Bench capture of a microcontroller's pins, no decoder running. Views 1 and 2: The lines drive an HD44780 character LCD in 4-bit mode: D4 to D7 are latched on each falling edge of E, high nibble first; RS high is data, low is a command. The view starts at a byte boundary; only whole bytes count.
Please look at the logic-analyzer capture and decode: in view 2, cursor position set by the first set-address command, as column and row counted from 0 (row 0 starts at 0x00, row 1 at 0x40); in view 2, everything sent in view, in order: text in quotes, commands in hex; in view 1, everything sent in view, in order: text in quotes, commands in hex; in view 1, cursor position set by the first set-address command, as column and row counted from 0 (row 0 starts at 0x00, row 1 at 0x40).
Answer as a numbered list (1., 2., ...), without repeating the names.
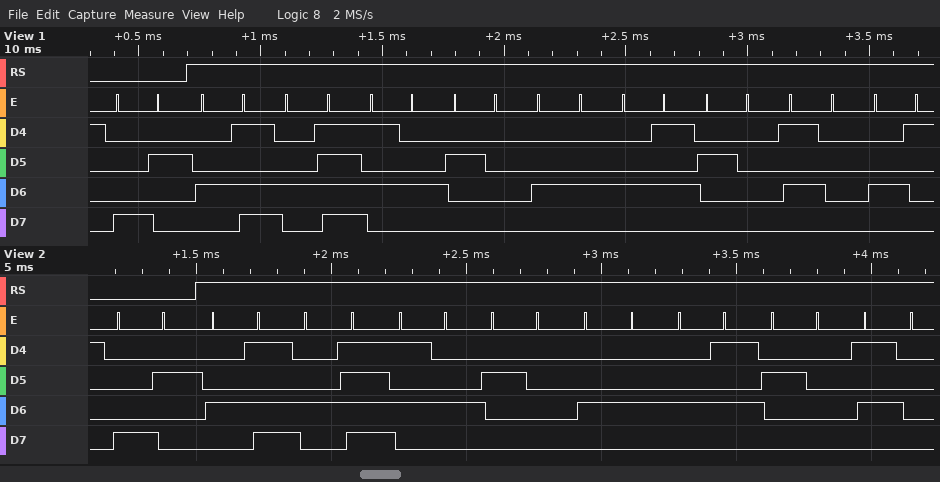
1. column 2, row 0
2. 0x82 "MOT DE P"
3. 0x82 "MOT DE PA"
4. column 2, row 0
